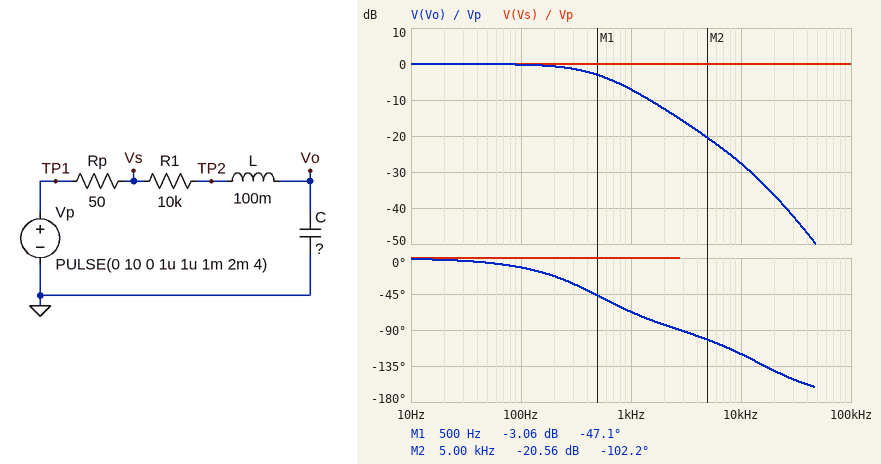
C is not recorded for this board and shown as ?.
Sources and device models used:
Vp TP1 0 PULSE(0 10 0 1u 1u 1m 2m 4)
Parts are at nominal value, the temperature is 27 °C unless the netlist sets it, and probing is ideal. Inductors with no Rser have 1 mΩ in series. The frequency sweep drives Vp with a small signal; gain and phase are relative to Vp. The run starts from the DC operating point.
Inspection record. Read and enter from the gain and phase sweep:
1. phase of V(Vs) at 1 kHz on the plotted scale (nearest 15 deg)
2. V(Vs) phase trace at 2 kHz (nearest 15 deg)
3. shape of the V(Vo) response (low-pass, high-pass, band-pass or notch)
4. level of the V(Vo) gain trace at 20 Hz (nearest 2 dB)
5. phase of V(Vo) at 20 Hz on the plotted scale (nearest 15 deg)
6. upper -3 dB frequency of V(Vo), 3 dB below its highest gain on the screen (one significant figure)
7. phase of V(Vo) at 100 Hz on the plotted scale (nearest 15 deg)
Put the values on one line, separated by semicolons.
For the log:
0 deg; 0 deg; low-pass; 0 dB; 0 deg; 500 Hz; -15 deg
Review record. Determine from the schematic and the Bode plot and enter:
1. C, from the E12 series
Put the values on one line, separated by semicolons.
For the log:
33 nF
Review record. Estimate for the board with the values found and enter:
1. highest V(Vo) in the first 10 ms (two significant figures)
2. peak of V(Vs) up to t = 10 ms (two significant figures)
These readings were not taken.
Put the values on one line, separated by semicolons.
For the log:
9.6 V; 10 V
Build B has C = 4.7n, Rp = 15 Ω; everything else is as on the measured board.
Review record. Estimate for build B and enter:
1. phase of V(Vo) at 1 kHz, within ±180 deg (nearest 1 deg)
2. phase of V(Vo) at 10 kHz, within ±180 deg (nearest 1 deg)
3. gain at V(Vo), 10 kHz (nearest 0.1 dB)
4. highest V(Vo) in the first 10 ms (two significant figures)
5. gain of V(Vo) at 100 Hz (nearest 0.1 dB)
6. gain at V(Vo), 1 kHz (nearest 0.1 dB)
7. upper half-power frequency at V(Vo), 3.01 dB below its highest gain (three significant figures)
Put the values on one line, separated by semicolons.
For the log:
-17 deg; -106 deg; -9.8 dB; 10 V; 0 dB; -0.2 dB; 4.21 kHz
